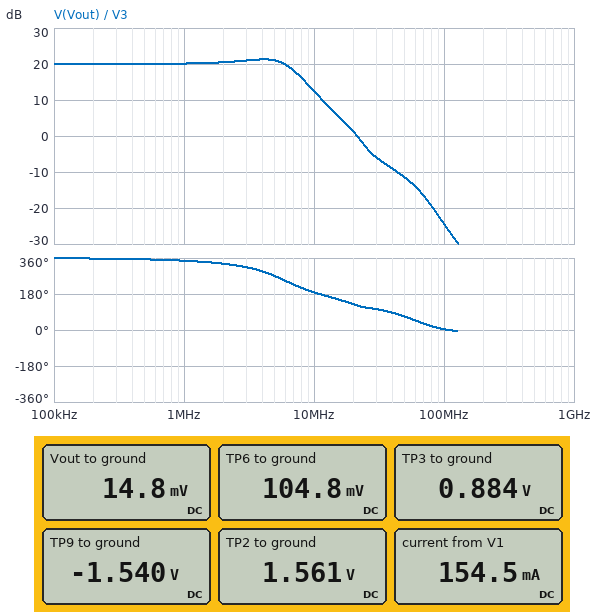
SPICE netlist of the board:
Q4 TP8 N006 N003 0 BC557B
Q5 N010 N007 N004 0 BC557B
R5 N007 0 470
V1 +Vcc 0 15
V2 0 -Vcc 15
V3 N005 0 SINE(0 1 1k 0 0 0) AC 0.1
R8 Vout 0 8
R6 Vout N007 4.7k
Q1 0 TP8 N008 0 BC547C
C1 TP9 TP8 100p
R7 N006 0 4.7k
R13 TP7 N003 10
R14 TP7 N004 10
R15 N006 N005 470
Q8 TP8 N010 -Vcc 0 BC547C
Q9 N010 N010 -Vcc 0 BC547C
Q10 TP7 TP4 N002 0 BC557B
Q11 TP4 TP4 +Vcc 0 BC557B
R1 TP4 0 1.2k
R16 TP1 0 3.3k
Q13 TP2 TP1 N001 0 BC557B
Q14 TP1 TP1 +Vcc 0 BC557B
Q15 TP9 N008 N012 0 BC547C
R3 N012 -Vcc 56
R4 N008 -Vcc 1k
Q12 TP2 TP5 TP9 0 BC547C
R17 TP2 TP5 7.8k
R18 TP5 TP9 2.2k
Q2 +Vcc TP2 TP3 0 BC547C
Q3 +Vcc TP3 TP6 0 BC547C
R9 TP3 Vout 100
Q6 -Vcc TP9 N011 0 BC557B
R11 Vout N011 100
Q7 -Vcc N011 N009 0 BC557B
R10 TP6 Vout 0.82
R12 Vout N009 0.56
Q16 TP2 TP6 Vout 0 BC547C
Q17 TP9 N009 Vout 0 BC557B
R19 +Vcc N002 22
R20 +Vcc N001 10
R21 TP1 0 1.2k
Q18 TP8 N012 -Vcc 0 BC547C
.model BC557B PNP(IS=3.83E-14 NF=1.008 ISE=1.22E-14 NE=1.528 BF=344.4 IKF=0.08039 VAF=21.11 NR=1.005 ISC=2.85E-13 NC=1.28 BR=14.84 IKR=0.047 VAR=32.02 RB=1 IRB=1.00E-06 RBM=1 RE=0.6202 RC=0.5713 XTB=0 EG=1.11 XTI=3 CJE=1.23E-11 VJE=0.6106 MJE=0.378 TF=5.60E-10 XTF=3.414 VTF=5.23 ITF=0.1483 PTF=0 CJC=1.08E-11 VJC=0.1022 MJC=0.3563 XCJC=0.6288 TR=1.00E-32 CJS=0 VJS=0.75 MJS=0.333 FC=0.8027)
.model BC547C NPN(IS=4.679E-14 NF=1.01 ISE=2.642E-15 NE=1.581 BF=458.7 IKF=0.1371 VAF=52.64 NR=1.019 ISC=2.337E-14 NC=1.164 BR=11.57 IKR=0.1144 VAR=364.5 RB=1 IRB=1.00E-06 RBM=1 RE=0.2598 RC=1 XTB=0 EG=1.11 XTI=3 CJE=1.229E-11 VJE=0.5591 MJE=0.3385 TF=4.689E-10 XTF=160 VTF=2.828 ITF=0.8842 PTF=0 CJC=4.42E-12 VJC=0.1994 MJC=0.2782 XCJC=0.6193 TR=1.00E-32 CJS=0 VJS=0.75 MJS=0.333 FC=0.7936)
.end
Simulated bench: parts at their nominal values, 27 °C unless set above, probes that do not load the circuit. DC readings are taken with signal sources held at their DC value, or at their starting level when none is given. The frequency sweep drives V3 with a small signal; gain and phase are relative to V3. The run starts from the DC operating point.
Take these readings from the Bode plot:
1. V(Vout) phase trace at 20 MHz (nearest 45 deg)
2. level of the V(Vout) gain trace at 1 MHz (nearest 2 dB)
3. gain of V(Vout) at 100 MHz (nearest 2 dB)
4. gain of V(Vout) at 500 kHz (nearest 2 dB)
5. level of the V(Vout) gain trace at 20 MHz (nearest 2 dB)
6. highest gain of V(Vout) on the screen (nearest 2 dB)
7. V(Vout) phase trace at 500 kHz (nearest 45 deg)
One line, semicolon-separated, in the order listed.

135 deg; 20 dB; -24 dB; 20 dB; 2 dB; 22 dB; 360 deg
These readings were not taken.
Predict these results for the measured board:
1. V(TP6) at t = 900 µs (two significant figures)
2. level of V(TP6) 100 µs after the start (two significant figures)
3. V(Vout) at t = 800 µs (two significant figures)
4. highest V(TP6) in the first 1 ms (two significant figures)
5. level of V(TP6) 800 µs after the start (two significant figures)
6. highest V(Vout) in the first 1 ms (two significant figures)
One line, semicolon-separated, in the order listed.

-5.9 V; 6.5 V; -9.5 V; 7.3 V; -9.5 V; 6.6 V
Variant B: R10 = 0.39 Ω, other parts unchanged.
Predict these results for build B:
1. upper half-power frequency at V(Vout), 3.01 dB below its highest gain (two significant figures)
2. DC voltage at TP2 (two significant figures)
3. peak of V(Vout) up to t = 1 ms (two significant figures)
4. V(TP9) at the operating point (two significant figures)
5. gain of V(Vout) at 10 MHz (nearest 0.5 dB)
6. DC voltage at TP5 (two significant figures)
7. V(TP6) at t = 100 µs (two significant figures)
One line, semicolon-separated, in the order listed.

7.0 MHz; 1.5 V; 10 V; -1.6 V; 13.0 dB; -910 mV; 6.2 V
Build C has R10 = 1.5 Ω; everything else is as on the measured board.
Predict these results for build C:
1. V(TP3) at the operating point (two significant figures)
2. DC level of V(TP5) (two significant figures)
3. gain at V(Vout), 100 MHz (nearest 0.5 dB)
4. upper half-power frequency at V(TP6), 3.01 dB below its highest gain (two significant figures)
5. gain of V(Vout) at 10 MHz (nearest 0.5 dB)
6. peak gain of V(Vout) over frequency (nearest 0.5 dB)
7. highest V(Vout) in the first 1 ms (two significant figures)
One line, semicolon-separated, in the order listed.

920 mV; -840 mV; -24.0 dB; 6.8 MHz; 12.0 dB; 21.0 dB; 3.7 V
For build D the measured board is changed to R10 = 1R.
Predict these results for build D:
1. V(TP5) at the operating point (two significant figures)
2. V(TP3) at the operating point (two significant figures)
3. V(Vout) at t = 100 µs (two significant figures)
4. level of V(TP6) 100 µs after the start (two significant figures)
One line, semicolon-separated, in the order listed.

-870 mV; 890 mV; 5.5 V; 6.1 V
